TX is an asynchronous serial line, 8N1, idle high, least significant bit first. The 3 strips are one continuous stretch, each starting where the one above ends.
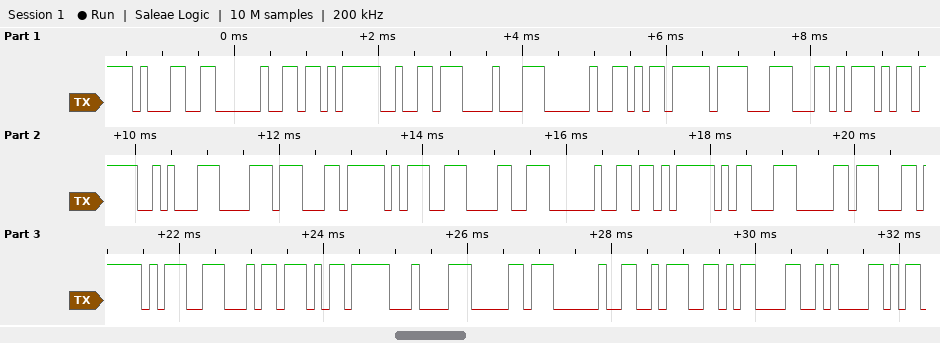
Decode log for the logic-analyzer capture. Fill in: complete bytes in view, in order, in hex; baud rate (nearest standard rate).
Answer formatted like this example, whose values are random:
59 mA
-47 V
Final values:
31 20 EB B2 88 20 ED 8F AC ED 8A B8 EC 9D 98 20 EB 8D B0 EC 9D B4 ED 84 B0 20 3A 0D 0A
9600 baud
